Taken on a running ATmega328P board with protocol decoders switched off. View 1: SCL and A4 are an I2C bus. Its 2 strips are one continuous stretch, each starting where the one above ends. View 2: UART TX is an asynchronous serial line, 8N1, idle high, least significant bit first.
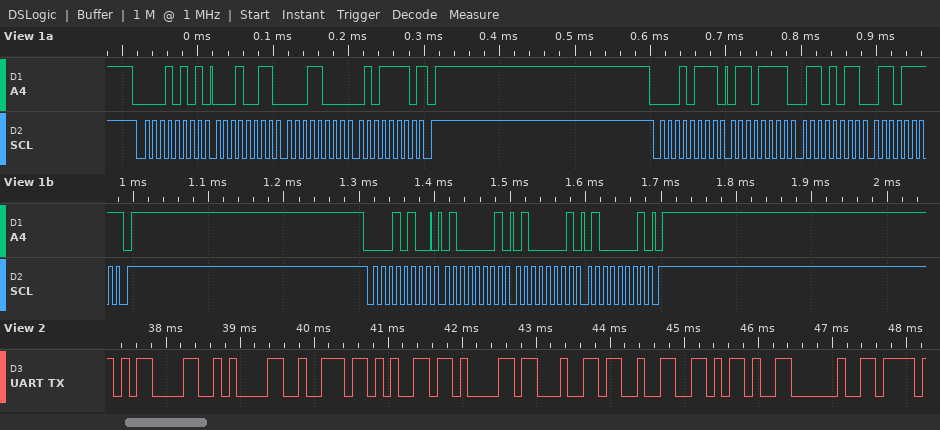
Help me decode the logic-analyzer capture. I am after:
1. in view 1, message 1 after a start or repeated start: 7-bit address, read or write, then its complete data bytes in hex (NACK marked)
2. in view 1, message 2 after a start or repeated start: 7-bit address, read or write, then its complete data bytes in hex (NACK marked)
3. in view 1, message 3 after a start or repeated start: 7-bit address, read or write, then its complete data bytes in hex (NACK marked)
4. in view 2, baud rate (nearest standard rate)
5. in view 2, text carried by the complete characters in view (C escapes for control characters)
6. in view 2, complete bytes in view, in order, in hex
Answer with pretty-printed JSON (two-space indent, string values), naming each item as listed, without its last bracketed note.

{
  "in view 1, message 1 after a start or repeated start: 7-bit address, read or write, then its complete data bytes in hex": "0x0A read: 13 18 5E NACK",
  "in view 1, message 2 after a start or repeated start: 7-bit address, read or write, then its complete data bytes in hex": "0x0B read: 6F 6B 6F NACK",
  "in view 1, message 3 after a start or repeated start: 7-bit address, read or write, then its complete data bytes in hex": "0x0A write: 41 41 41",
  "in view 2, baud rate": "9600 baud",
  "in view 2, text carried by the complete characters in view": "\"\\r\\nread2- \"",
  "in view 2, complete bytes in view, in order, in hex": "0D 0A 72 65 61 64 32 2D 20"
}
